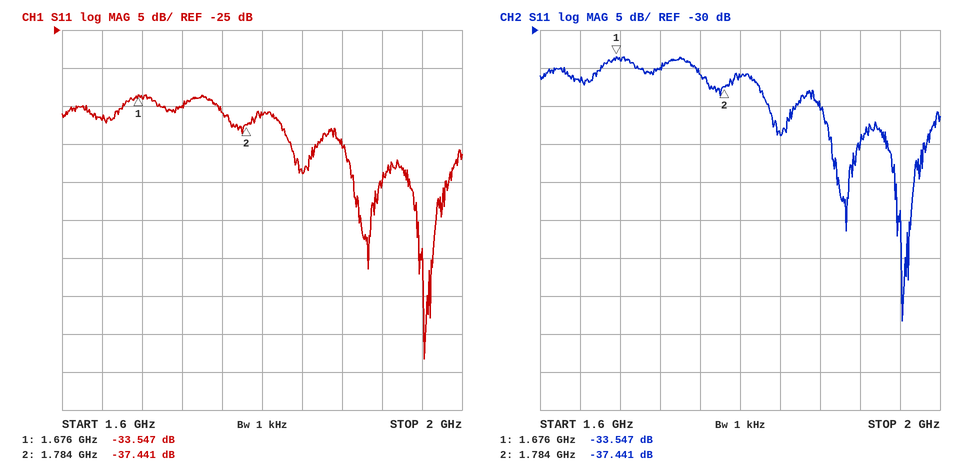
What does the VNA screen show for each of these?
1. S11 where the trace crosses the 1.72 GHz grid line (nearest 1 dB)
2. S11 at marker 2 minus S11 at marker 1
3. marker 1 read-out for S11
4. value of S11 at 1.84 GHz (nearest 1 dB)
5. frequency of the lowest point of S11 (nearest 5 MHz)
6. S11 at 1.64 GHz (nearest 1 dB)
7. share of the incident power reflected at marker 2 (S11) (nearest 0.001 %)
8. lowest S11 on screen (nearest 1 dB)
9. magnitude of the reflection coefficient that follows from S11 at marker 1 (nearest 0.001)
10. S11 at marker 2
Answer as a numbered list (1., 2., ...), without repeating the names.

1. -35 dB
2. -3.894 dB
3. -33.547 dB
4. -44 dB
5. 1.960 GHz
6. -37 dB
7. 0.018 %
8. -68 dB
9. 0.021
10. -37.441 dB
